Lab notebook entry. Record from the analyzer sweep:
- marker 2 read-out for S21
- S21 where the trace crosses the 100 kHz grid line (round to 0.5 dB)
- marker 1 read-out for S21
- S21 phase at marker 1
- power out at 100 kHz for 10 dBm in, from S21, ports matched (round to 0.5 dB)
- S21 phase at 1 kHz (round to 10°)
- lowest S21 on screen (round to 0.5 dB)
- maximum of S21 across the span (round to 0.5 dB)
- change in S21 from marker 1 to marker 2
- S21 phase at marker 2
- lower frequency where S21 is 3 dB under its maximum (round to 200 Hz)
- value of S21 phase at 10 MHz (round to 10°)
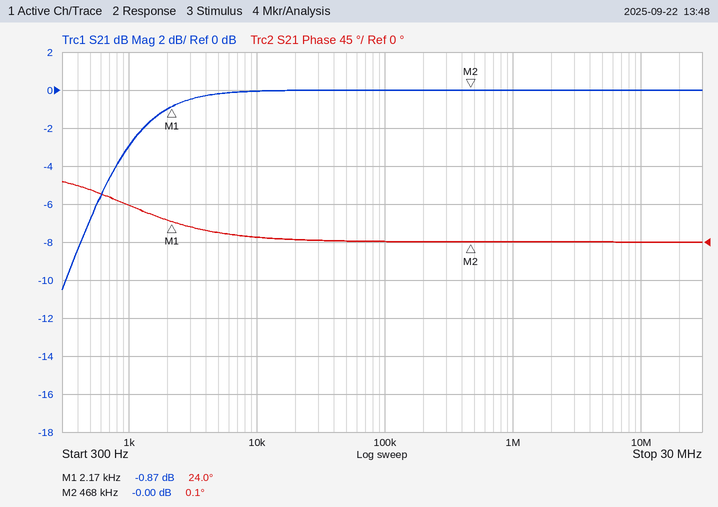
-0.00 dB
0.0 dB
-0.87 dB
24.0°
10.0 dBm
40°
-10.5 dB
0.0 dB
0.87 dB
0.1°
1.0 kHz
0°
